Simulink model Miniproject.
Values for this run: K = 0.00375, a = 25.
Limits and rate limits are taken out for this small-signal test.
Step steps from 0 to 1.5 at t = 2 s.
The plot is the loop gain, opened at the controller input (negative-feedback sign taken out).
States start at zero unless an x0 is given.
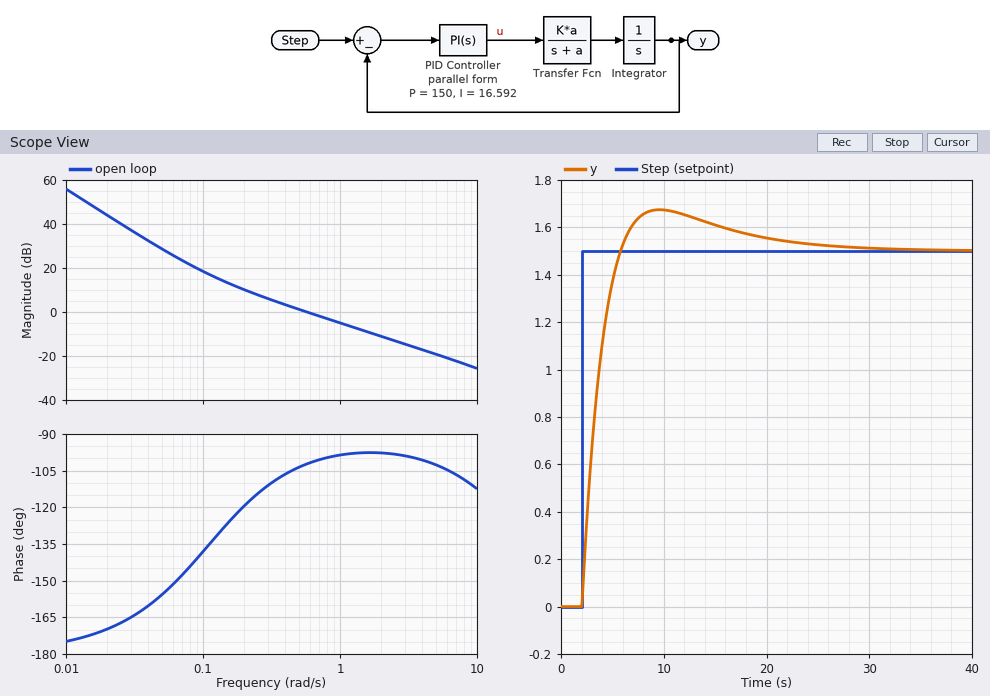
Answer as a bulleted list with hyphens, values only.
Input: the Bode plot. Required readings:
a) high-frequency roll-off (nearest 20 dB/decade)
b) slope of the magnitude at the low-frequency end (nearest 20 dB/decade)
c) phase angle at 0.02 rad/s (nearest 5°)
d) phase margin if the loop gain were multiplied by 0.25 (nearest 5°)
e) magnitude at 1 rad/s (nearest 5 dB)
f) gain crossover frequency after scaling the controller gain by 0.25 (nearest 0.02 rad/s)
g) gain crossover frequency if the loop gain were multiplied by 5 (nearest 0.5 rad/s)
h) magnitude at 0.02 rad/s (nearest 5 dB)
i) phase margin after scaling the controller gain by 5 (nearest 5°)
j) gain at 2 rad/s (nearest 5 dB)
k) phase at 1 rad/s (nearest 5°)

- -20 dB/decade
- -40 dB/decade
- -170°
- 55°
- -5 dB
- 0.16 rad/s
- 3.0 rad/s
- 45 dB
- 80°
- -10 dB
- -100°
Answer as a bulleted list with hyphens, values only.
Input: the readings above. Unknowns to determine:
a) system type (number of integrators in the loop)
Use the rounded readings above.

- 2
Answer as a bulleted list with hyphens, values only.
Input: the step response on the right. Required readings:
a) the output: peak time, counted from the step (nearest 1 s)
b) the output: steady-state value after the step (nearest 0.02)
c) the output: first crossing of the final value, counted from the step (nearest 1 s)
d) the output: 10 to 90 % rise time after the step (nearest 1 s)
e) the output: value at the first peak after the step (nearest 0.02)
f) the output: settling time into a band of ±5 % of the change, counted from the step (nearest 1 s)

- 8 s
- 1.50
- 4 s
- 3 s
- 1.68
- 16 s
